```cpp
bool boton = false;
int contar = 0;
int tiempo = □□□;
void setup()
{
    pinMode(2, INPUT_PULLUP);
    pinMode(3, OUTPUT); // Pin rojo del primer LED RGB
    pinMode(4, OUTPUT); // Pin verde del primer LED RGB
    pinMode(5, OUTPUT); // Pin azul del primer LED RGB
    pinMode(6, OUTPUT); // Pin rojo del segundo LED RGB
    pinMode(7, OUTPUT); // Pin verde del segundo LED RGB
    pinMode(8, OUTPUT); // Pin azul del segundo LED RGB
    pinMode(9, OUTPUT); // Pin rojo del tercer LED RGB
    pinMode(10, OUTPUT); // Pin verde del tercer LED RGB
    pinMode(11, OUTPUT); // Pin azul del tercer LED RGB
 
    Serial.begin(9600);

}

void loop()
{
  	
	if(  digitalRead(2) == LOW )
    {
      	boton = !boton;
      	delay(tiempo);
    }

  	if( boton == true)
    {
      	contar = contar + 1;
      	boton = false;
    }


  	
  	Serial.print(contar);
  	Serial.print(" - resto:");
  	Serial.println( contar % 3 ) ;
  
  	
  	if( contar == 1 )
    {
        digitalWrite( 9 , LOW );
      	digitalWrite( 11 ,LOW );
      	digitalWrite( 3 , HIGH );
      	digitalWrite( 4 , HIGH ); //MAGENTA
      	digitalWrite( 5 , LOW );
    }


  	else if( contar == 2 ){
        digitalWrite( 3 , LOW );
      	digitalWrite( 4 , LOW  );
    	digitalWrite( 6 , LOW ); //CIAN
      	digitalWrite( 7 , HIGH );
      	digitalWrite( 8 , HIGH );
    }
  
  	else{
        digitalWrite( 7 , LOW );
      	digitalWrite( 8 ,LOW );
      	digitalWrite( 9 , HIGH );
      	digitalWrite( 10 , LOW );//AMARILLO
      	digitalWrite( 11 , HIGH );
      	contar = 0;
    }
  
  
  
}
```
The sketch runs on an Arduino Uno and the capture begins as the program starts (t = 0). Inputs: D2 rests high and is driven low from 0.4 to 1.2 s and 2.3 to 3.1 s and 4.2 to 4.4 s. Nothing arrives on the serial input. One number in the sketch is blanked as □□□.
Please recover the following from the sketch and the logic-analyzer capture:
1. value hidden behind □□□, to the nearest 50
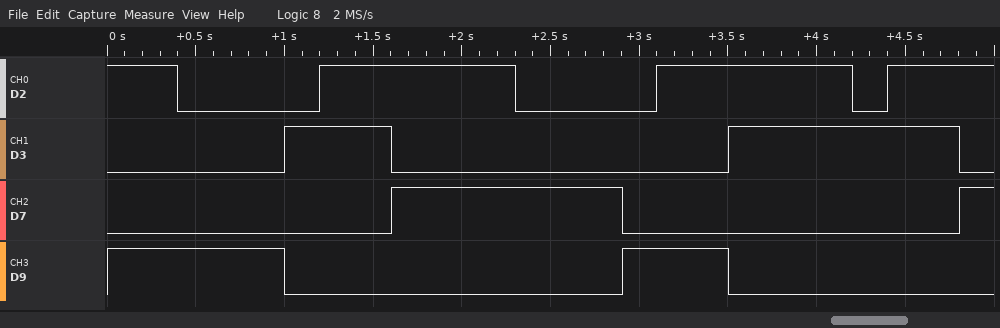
600
